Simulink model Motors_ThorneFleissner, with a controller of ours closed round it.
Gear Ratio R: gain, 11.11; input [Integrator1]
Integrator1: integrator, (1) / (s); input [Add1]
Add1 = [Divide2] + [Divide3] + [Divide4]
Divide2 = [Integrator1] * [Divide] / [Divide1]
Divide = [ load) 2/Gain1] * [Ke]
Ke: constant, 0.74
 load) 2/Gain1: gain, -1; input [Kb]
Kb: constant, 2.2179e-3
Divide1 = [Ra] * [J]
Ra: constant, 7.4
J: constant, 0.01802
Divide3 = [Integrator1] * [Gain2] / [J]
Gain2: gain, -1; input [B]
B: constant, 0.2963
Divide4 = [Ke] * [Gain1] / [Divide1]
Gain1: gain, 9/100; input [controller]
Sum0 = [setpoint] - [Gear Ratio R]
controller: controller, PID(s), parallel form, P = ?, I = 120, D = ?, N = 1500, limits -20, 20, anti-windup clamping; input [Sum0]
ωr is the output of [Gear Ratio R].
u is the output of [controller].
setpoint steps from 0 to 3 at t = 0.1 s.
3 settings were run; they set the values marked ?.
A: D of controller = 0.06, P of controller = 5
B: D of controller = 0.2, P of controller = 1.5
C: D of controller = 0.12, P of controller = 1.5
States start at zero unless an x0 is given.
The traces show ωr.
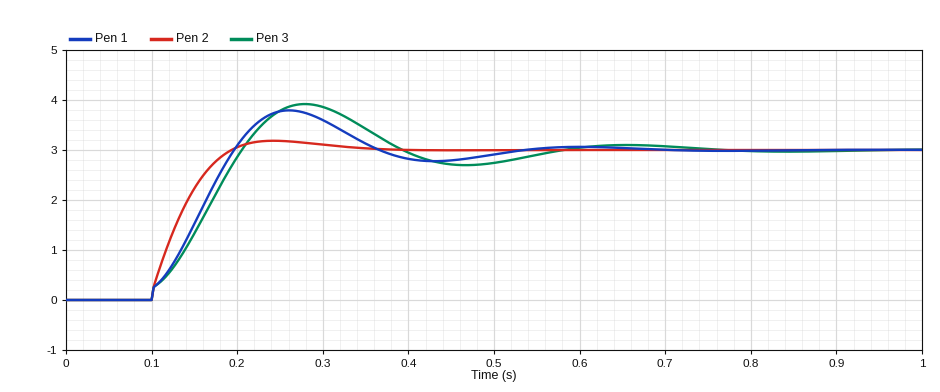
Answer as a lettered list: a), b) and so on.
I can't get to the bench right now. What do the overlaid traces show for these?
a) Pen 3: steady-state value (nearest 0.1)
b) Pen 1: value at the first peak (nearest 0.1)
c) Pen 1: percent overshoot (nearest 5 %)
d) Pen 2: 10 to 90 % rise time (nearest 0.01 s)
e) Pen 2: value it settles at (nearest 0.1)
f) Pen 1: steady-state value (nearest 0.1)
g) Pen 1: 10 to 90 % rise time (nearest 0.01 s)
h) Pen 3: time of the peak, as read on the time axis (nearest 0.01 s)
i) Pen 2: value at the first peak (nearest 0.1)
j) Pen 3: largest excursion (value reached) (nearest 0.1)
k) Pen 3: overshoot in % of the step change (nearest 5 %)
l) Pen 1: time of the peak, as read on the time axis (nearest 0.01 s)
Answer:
a) 3.0
b) 3.8
c) 25 %
d) 0.07 s
e) 3.0
f) 3.0
g) 0.08 s
h) 0.28 s
i) 3.2
j) 3.9
k) 30 %
l) 0.26 s
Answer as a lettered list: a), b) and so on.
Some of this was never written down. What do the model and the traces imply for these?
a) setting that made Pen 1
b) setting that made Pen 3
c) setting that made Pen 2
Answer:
a) C
b) B
c) A
